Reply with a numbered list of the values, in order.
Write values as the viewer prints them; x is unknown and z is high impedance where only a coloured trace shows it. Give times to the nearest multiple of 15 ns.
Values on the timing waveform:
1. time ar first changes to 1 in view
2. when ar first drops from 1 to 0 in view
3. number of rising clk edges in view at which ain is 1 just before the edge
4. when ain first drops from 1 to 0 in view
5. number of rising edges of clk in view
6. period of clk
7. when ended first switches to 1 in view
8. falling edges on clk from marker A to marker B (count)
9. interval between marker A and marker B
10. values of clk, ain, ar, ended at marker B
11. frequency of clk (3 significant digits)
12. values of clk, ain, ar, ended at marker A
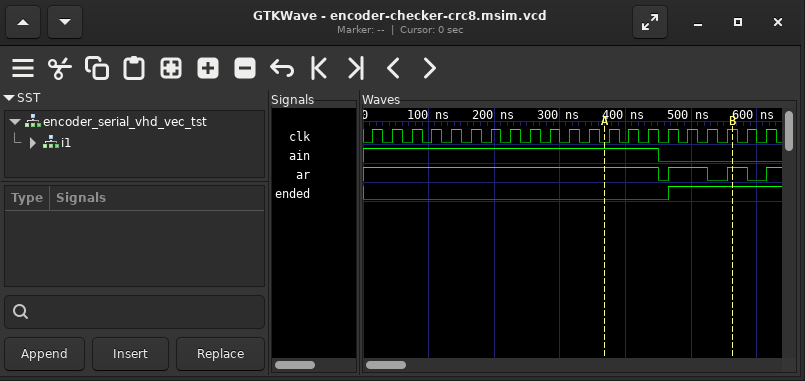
1. 465 ns
2. 450 ns
3. 15
4. 450 ns
5. 21
6. 30 ns
7. 465 ns
8. 6
9. 195 ns
10. clk=1, ain=0, ar=1, ended=1
11. 33.3 MHz
12. clk=0, ain=1, ar=1, ended=0
